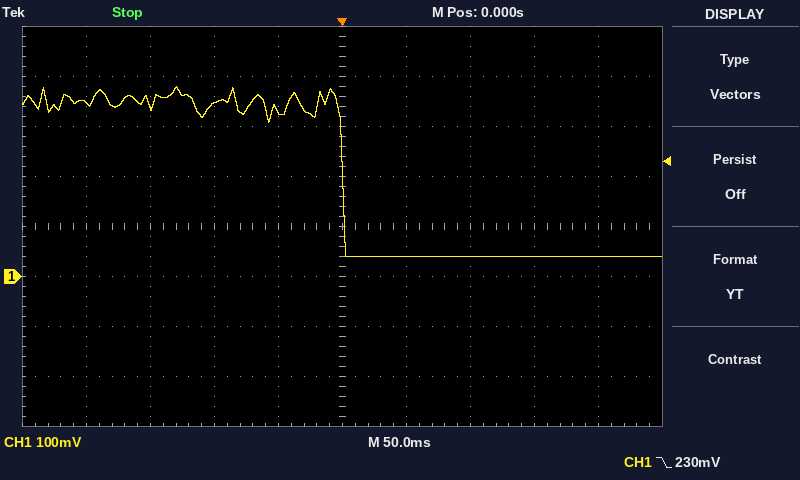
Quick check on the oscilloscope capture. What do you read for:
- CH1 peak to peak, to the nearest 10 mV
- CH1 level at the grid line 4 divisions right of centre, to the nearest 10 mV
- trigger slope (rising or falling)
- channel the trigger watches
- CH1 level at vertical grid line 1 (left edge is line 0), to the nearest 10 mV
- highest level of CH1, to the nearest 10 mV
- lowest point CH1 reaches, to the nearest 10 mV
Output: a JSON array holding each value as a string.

["340 mV", "40 mV", "falling", "CH1", "350 mV", "380 mV", "40 mV"]
